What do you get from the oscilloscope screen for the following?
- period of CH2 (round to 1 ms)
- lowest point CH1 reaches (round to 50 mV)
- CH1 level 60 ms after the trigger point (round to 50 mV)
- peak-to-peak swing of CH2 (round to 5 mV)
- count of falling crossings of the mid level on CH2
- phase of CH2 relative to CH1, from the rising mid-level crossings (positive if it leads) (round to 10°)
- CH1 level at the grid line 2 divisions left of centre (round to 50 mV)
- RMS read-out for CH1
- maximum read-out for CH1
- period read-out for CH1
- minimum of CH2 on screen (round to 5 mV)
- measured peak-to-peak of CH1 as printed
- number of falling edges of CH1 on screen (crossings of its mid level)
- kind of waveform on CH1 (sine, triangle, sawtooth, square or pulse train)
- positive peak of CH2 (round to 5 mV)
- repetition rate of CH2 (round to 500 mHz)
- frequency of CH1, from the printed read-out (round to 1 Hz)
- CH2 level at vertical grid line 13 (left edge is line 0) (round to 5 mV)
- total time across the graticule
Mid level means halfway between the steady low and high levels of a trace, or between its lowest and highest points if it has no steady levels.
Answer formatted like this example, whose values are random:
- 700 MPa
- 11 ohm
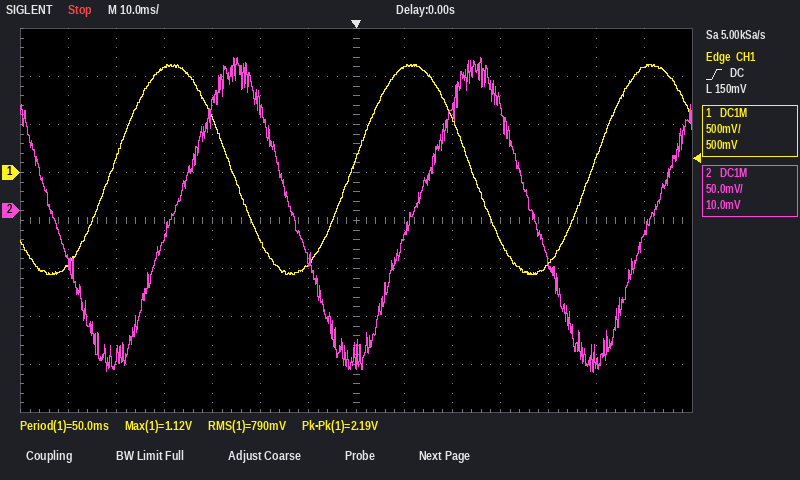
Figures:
- 50 ms
- -1.05 V
- 1.10 V
- 330 mV
- 3
- -90°
- -700 mV
- 790 mV
- 1.12 V
- 50.0 ms
- -170 mV
- 2.19 V
- 2
- sine
- 160 mV
- 20.0 Hz
- 20 Hz
- -25 mV
- 140 ms
